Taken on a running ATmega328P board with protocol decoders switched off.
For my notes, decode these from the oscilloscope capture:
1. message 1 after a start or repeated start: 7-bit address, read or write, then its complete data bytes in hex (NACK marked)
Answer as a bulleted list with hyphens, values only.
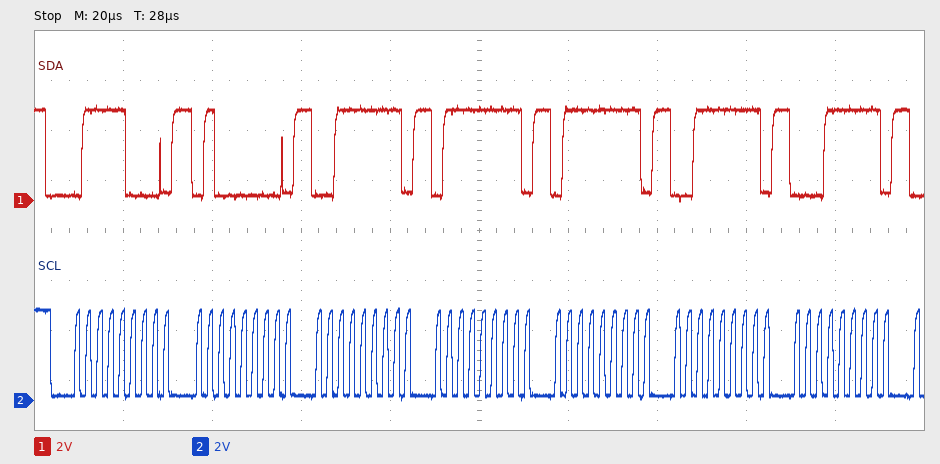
- 0x3C write: 40 3F 7F 7F 3F 1F
